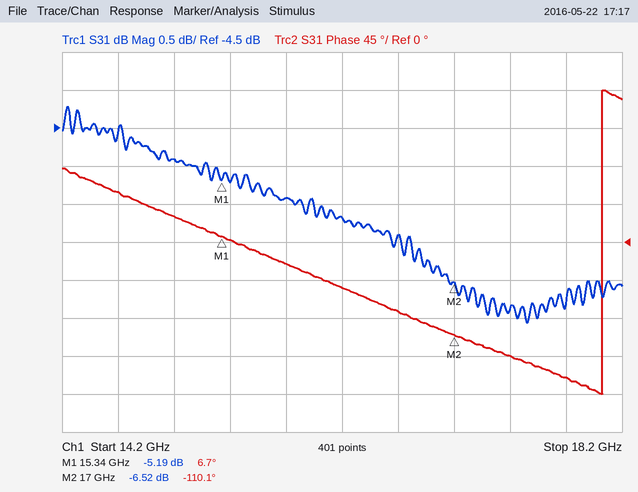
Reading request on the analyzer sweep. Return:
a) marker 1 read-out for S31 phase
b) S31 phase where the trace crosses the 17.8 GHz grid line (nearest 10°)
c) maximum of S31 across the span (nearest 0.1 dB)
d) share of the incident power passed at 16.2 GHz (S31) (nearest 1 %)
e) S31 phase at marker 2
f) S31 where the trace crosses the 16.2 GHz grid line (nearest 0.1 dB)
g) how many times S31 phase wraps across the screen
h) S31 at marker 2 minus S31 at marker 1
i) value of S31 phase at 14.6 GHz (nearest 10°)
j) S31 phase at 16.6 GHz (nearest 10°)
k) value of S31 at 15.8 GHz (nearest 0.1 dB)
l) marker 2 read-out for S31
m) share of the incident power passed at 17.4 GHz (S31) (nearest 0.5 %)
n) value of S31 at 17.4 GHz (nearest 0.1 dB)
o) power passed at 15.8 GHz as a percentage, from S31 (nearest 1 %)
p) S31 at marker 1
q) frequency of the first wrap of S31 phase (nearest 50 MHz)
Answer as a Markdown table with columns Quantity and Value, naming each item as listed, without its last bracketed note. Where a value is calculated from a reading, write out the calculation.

| Quantity | Value |
|---|---|
| marker 1 read-out for S31 phase | 6.7° |
| S31 phase where the trace crosses the 17.8 GHz grid line | -160° |
| maximum of S31 across the span | -4.2 dB |
| share of the incident power passed at 16.2 GHz (S31) | 10^(-5.7/10) ≈ 27 % |
| S31 phase at marker 2 | -110.1° |
| S31 where the trace crosses the 16.2 GHz grid line | -5.7 dB |
| how many times S31 phase wraps across the screen | 1 |
| S31 at marker 2 minus S31 at marker 1 | -6.52 − (-5.19) = -1.33 dB |
| value of S31 phase at 14.6 GHz | 60° |
| S31 phase at 16.6 GHz | -80° |
| value of S31 at 15.8 GHz | -5.4 dB |
| marker 2 read-out for S31 | -6.52 dB |
| share of the incident power passed at 17.4 GHz (S31) | 10^(-6.9/10) ≈ 20.4 %, so 20.5 % to the nearest 0.5 % |
| value of S31 at 17.4 GHz | -6.9 dB |
| power passed at 15.8 GHz as a percentage, from S31 | 10^(-5.4/10) ≈ 29 % |
| S31 at marker 1 | -5.19 dB |
| frequency of the first wrap of S31 phase | 18.05 GHz |
